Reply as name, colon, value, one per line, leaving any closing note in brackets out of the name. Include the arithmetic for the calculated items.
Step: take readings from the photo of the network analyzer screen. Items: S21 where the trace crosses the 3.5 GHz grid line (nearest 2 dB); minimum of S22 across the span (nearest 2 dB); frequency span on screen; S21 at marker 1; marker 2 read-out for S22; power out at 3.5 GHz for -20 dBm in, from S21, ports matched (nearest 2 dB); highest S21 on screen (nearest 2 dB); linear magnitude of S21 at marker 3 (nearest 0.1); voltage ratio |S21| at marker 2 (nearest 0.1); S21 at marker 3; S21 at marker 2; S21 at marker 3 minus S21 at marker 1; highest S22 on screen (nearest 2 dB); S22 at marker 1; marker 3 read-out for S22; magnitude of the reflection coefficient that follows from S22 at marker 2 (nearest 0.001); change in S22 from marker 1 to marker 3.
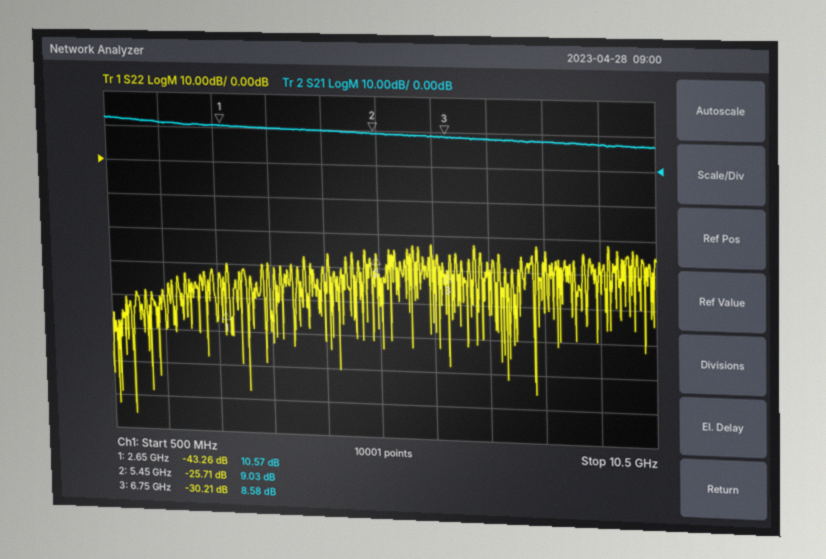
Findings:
S21 where the trace crosses the 3.5 GHz grid line: 10 dB
minimum of S22 across the span: -76 dB
frequency span on screen: 10 GHz
S21 at marker 1: 10.57 dB
marker 2 read-out for S22: -25.71 dB
power out at 3.5 GHz for -20 dBm in, from S21, ports matched: -20 dBm + (10 dB) = -10 dBm
highest S21 on screen: 12 dB
linear magnitude of S21 at marker 3: 10^(8.58/20) ≈ 2.7
voltage ratio |S21| at marker 2: 10^(9.03/20) ≈ 2.8
S21 at marker 3: 8.58 dB
S21 at marker 2: 9.03 dB
S21 at marker 3 minus S21 at marker 1: 8.58 − (10.57) = -1.99 dB
highest S22 on screen: -22 dB
S22 at marker 1: -43.26 dB
marker 3 read-out for S22: -30.21 dB
magnitude of the reflection coefficient that follows from S22 at marker 2: 10^(-25.71/20) ≈ 0.052
change in S22 from marker 1 to marker 3: -30.21 − (-43.26) = 13.05 dB
